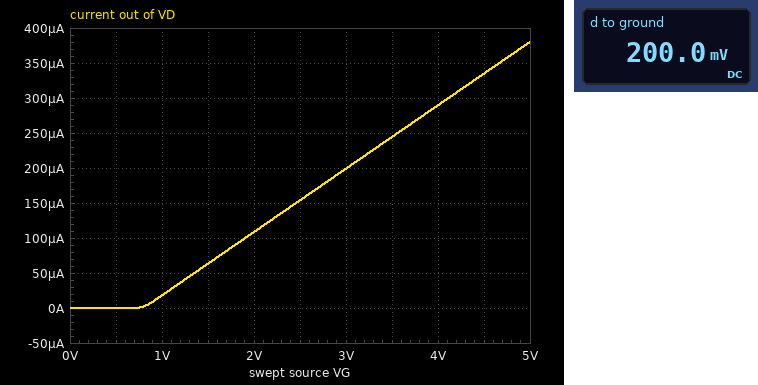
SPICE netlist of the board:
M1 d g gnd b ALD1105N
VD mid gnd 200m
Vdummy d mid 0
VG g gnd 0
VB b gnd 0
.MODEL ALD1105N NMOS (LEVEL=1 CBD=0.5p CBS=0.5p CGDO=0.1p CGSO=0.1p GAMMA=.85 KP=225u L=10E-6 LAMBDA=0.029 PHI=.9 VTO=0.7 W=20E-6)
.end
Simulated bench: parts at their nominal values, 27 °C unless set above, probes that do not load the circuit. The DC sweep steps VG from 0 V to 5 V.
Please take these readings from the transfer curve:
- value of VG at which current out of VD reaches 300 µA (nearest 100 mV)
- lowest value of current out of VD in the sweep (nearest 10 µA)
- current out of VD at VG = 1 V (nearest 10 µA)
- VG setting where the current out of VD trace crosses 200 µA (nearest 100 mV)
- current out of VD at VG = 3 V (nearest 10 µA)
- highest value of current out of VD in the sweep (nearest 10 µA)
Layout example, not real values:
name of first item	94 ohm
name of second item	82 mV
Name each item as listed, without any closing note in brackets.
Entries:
value of VG at which current out of VD reaches 300 µA	4.1 V
lowest value of current out of VD in the sweep	0 A
current out of VD at VG = 1 V	20 µA
VG setting where the current out of VD trace crosses 200 µA	3.0 V
current out of VD at VG = 3 V	200 µA
highest value of current out of VD in the sweep	380 µA
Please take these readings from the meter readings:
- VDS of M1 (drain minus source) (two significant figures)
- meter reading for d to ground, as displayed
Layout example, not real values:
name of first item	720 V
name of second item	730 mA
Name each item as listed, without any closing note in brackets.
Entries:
VDS of M1 (drain minus source)	200 mV
meter reading for d to ground, as displayed	200.0 mV
